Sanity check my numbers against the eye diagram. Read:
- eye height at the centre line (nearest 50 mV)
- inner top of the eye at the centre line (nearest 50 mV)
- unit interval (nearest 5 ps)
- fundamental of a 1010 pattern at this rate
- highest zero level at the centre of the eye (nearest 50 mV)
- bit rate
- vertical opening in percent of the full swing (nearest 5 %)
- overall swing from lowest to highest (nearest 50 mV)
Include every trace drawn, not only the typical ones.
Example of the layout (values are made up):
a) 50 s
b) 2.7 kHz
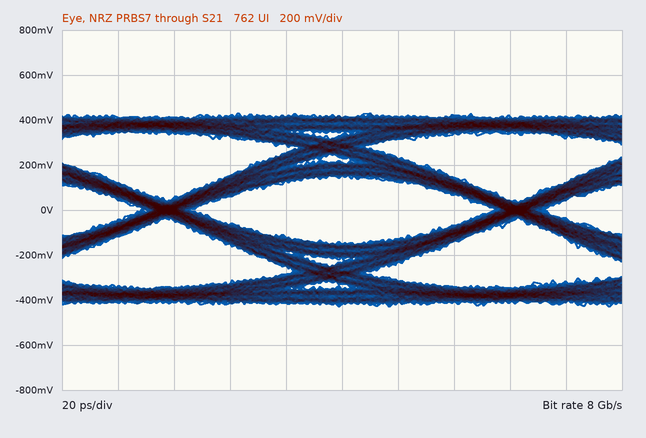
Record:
a) 300 mV
b) 150 mV
c) 125 ps
d) 4 GHz
e) -150 mV
f) 8 Gb/s
g) 35 %
h) 850 mV
